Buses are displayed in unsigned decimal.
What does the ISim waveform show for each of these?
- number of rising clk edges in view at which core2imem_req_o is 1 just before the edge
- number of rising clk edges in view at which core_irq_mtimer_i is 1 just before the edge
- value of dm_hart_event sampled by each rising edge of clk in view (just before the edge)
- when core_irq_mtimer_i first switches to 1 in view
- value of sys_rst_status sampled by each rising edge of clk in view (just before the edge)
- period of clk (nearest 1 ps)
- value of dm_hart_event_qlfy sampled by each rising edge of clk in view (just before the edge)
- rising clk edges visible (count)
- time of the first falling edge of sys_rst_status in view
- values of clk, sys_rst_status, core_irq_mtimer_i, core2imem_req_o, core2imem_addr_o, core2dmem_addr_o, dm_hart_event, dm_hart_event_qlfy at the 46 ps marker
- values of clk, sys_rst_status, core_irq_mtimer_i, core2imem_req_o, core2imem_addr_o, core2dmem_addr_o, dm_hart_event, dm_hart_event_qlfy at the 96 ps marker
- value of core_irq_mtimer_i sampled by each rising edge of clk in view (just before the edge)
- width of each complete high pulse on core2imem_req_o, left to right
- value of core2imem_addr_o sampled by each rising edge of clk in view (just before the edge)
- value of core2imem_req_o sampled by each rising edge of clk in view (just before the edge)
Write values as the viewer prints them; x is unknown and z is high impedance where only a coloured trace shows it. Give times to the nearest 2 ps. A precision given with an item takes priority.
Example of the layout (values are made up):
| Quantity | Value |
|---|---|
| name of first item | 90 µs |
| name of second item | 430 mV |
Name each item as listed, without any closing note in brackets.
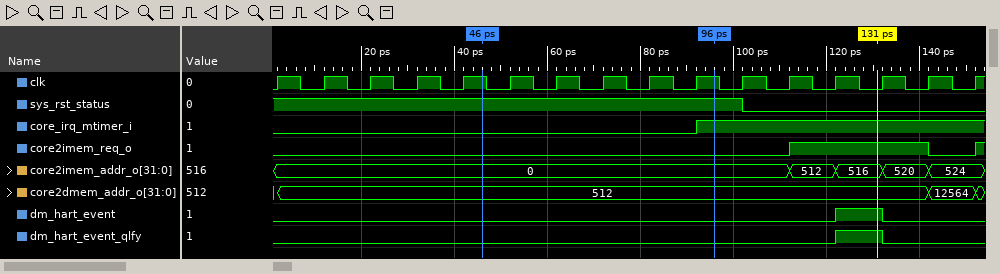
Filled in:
| Quantity | Value |
|---|---|
| number of rising clk edges in view at which core2imem_req_o is 1 just before the edge | 3 |
| number of rising clk edges in view at which core_irq_mtimer_i is 1 just before the edge | 6 |
| value of dm_hart_event sampled by each rising edge of clk in view | 0 0 0 0 0 0 0 0 0 0 0 0 0 1 0 0 |
| when core_irq_mtimer_i first switches to 1 in view | 92 ps |
| value of sys_rst_status sampled by each rising edge of clk in view | 1 1 1 1 1 1 1 1 1 1 1 0 0 0 0 0 |
| period of clk | 10 ps |
| value of dm_hart_event_qlfy sampled by each rising edge of clk in view | 0 0 0 0 0 0 0 0 0 0 0 0 0 1 0 0 |
| rising clk edges visible | 16 |
| time of the first falling edge of sys_rst_status in view | 102 ps |
| values of clk, sys_rst_status, core_irq_mtimer_i, core2imem_req_o, core2imem_addr_o, core2dmem_addr_o, dm_hart_event, dm_hart_event_qlfy at the 46 ps marker | clk=1, sys_rst_status=1, core_irq_mtimer_i=0, core2imem_req_o=0, core2imem_addr_o=0, core2dmem_addr_o=512, dm_hart_event=0, dm_hart_event_qlfy=0 |
| values of clk, sys_rst_status, core_irq_mtimer_i, core2imem_req_o, core2imem_addr_o, core2dmem_addr_o, dm_hart_event, dm_hart_event_qlfy at the 96 ps marker | clk=1, sys_rst_status=1, core_irq_mtimer_i=1, core2imem_req_o=0, core2imem_addr_o=0, core2dmem_addr_o=512, dm_hart_event=0, dm_hart_event_qlfy=0 |
| value of core_irq_mtimer_i sampled by each rising edge of clk in view | 0 0 0 0 0 0 0 0 0 0 1 1 1 1 1 1 |
| width of each complete high pulse on core2imem_req_o, left to right | 30 ps |
| value of core2imem_addr_o sampled by each rising edge of clk in view | 0, 0, 0, 0, 0, 0, 0, 0, 0, 0, 0, 0, 512, 516, 520, 524 |
| value of core2imem_req_o sampled by each rising edge of clk in view | 0 0 0 0 0 0 0 0 0 0 0 0 1 1 1 0 |
